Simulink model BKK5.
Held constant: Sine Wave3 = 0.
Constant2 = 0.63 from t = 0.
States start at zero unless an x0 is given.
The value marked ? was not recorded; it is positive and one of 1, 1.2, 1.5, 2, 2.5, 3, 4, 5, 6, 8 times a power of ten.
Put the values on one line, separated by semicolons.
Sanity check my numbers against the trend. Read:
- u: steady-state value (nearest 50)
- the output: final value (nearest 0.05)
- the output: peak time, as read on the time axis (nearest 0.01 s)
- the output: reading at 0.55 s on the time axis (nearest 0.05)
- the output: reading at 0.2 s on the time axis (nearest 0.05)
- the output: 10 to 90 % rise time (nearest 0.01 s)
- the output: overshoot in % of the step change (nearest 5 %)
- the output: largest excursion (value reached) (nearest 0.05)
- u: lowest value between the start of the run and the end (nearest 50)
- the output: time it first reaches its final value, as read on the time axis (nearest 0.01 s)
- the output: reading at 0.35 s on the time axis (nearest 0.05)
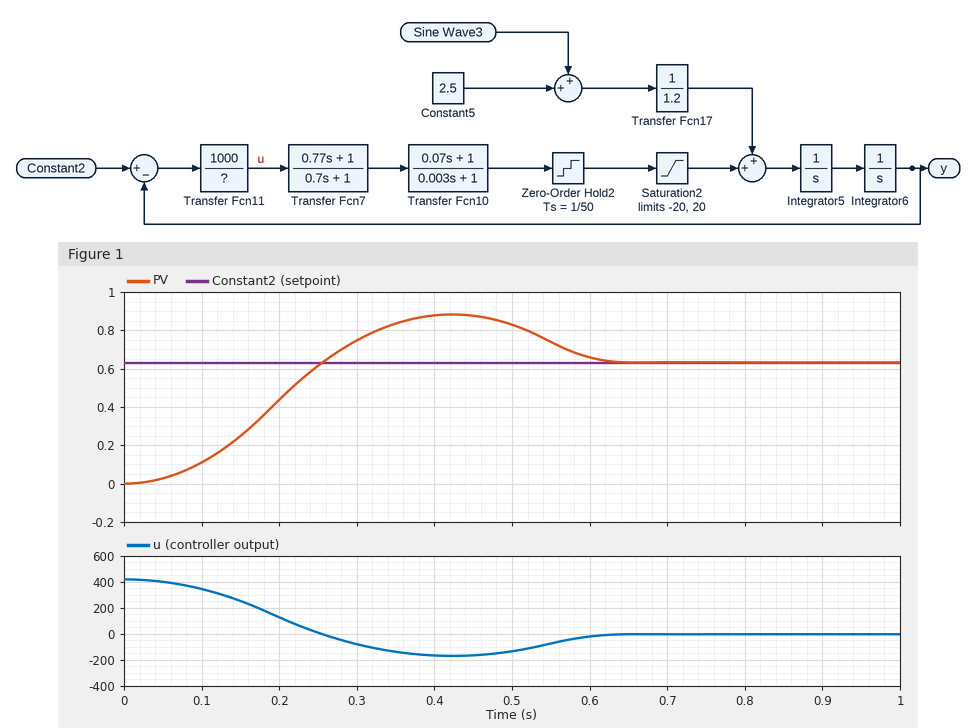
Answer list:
0; 0.65; 0.42 s; 0.75; 0.45; 0.16 s; 40 %; 0.90; -150; 0.26 s; 0.85
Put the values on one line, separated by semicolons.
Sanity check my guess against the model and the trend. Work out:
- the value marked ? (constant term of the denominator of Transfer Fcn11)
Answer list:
1.5
